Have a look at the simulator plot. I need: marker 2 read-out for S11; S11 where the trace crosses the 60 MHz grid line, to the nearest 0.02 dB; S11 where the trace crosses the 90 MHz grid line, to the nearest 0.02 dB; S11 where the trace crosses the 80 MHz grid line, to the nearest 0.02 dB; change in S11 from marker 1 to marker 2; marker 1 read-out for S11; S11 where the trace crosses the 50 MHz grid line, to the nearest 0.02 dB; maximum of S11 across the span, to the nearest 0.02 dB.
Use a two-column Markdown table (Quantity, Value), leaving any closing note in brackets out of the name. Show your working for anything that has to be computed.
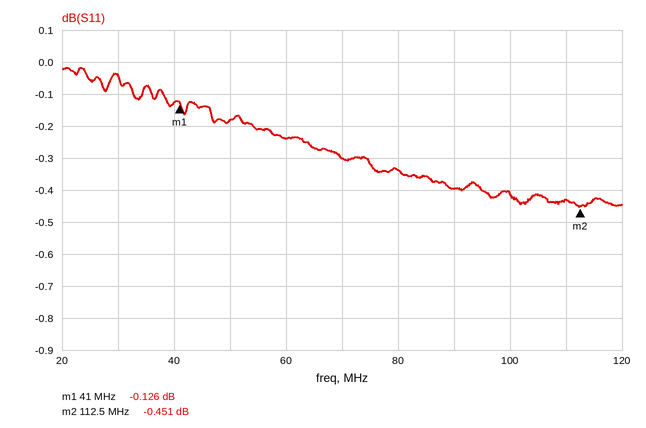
| Quantity | Value |
|---|---|
| marker 2 read-out for S11 | -0.451 dB |
| S11 where the trace crosses the 60 MHz grid line, to the nearest 0.02 dB | -0.24 dB |
| S11 where the trace crosses the 90 MHz grid line, to the nearest 0.02 dB | -0.40 dB |
| S11 where the trace crosses the 80 MHz grid line, to the nearest 0.02 dB | -0.34 dB |
| change in S11 from marker 1 to marker 2 | -0.451 − (-0.126) = -0.325 dB |
| marker 1 read-out for S11 | -0.126 dB |
| S11 where the trace crosses the 50 MHz grid line, to the nearest 0.02 dB | -0.18 dB |
| maximum of S11 across the span, to the nearest 0.02 dB | -0.02 dB |
